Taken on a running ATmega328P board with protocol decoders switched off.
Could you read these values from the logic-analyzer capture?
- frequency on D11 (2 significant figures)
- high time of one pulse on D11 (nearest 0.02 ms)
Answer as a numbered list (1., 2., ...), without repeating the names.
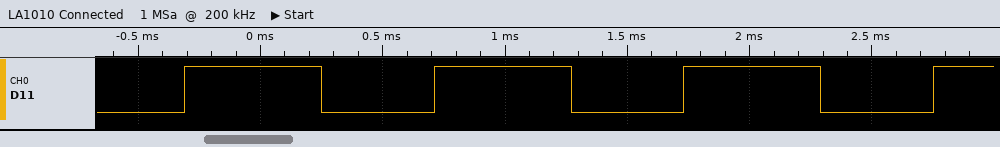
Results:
1. 980 Hz
2. 0.56 ms
